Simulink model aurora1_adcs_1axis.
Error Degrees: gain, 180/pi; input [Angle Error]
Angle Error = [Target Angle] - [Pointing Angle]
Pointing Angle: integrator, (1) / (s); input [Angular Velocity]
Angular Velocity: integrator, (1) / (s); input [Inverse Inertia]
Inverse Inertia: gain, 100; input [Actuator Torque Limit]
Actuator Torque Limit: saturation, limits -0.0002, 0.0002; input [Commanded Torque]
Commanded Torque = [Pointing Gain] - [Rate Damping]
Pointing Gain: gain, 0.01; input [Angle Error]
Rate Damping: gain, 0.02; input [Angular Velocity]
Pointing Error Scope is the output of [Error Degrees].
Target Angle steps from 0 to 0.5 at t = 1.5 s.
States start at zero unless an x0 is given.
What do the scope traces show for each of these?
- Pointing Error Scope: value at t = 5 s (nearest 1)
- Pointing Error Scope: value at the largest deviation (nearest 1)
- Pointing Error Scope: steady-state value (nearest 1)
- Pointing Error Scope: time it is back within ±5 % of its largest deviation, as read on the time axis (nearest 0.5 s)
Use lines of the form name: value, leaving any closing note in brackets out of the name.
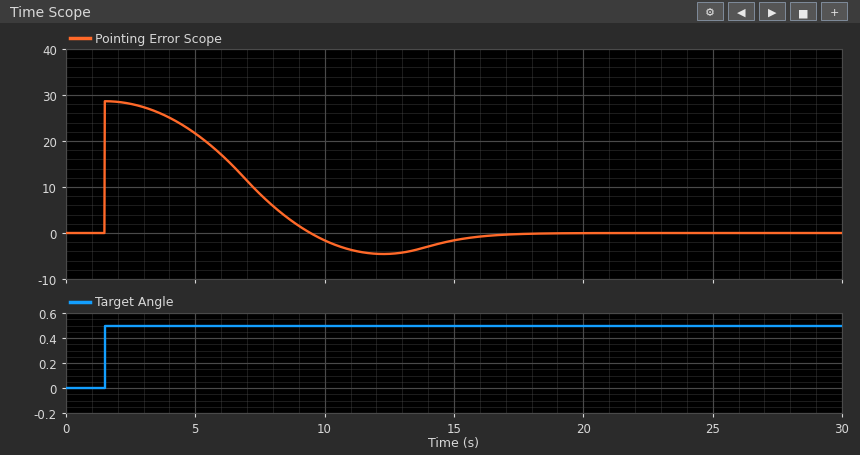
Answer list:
Pointing Error Scope: value at t = 5 s: 22
Pointing Error Scope: value at the largest deviation: 29
Pointing Error Scope: steady-state value: 0
Pointing Error Scope: time it is back within ±5 % of its largest deviation, as read on the time axis: 15.0 s
